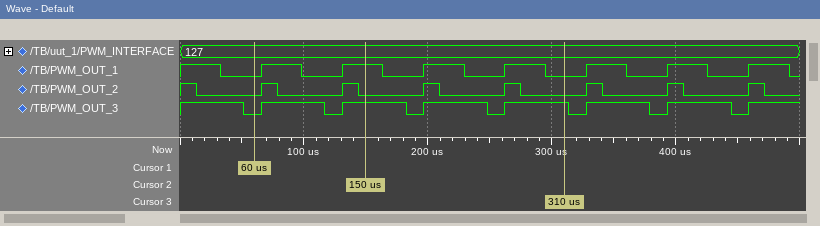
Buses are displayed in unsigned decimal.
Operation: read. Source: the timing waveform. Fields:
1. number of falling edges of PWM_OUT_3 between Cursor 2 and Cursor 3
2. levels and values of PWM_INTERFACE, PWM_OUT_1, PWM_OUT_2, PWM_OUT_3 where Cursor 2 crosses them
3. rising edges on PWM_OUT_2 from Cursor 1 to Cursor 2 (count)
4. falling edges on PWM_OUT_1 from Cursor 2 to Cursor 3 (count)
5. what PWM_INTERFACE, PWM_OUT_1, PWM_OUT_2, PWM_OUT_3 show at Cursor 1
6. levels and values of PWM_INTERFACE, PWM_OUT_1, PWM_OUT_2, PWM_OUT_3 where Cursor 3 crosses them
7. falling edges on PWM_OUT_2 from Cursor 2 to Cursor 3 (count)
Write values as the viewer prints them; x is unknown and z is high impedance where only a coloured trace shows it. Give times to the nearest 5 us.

2
PWM_INTERFACE=127, PWM_OUT_1=1, PWM_OUT_2=0, PWM_OUT_3=1
2
3
PWM_INTERFACE=127, PWM_OUT_1=0, PWM_OUT_2=0, PWM_OUT_3=0
PWM_INTERFACE=127, PWM_OUT_1=0, PWM_OUT_2=0, PWM_OUT_3=1
2
